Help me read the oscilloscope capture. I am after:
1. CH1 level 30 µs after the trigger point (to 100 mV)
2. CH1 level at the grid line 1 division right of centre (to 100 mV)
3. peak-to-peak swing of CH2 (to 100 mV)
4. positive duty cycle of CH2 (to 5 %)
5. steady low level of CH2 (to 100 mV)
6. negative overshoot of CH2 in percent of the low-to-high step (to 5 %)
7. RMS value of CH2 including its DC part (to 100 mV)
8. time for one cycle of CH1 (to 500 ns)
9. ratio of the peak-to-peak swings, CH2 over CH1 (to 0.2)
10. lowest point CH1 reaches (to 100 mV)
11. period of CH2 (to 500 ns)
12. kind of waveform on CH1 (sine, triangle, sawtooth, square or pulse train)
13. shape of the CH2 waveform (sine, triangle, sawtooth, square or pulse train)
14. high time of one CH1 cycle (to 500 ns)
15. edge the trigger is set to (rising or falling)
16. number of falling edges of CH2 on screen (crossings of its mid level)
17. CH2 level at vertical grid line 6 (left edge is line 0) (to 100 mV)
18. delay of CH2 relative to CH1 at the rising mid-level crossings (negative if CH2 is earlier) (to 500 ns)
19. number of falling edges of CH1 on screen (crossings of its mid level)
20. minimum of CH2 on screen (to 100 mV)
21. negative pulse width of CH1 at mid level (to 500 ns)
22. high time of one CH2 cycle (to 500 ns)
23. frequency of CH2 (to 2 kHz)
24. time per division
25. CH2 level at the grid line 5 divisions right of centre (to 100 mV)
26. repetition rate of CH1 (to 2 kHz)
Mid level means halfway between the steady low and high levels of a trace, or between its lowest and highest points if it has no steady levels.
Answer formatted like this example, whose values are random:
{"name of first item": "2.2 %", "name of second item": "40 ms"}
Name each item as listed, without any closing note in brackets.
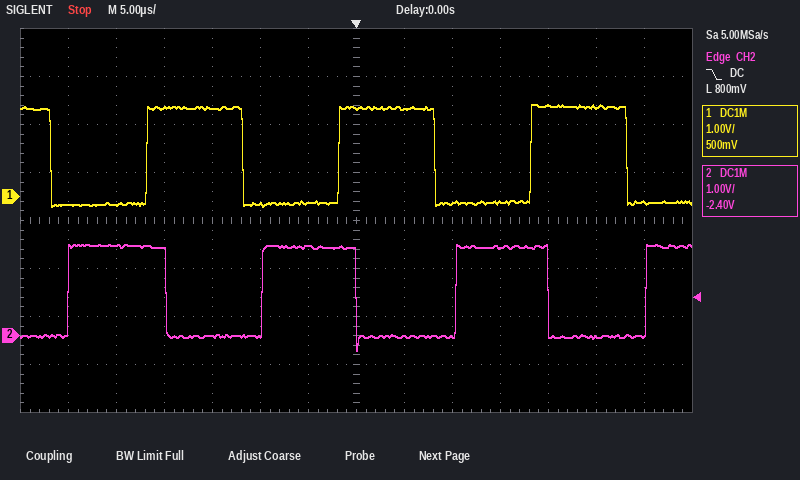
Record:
{"CH1 level 30 µs after the trigger point": "-100 mV", "CH1 level at the grid line 1 division right of centre": "1.8 V", "peak-to-peak swing of CH2": "2.2 V", "positive duty cycle of CH2": "50 %", "steady low level of CH2": "0.0 V", "negative overshoot of CH2 in percent of the low-to-high step": "15 %", "RMS value of CH2 including its DC part": "1.3 V", "time for one cycle of CH1": "20.0 µs", "ratio of the peak-to-peak swings, CH2 over CH1": "1.0", "lowest point CH1 reaches": "-200 mV", "period of CH2": "20.0 µs", "kind of waveform on CH1": "square", "shape of the CH2 waveform": "square", "high time of one CH1 cycle": "10.0 µs", "edge the trigger is set to": "falling", "number of falling edges of CH2 on screen": "3", "CH2 level at vertical grid line 6 (left edge is line 0)": "1.9 V", "delay of CH2 relative to CH1 at the rising mid-level crossings (negative if CH2 is earlier)": "-8.0 µs", "number of falling edges of CH1 on screen": "4", "minimum of CH2 on screen": "-300 mV", "negative pulse width of CH1 at mid level": "10.0 µs", "high time of one CH2 cycle": "10.0 µs", "frequency of CH2": "50 kHz", "time per division": "5 µs", "CH2 level at the grid line 5 divisions right of centre": "0.0 V", "repetition rate of CH1": "50 kHz"}
